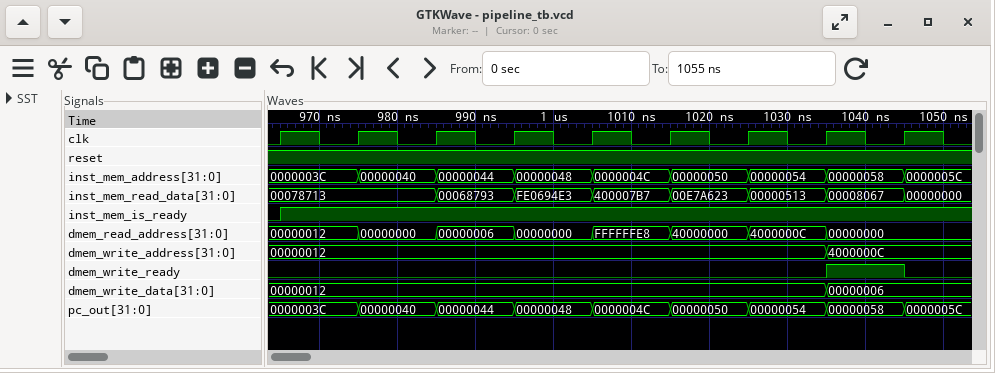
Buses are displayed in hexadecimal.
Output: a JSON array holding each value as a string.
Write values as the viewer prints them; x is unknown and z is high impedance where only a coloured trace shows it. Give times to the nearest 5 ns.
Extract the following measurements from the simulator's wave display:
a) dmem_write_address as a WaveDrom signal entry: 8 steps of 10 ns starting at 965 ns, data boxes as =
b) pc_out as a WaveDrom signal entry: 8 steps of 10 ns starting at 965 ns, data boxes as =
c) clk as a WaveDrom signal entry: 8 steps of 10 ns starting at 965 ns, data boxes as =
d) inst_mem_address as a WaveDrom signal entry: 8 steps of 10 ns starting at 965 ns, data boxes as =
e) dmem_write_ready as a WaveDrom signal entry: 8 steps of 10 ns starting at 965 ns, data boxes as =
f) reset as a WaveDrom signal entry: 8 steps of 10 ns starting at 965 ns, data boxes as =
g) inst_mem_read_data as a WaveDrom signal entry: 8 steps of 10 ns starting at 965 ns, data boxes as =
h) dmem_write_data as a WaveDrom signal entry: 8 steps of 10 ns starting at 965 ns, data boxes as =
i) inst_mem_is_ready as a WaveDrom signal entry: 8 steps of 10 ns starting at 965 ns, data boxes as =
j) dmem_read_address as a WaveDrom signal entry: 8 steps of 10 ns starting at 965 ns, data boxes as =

["{name: 'dmem_write_address', wave: '=......=', data: '00000012 4000000C'}", "{name: 'pc_out', wave: '========', data: '0000003C 00000040 00000044 00000048 0000004C 00000050 00000054 00000058'}", "{name: 'clk', wave: 'p.......'}", "{name: 'inst_mem_address', wave: '========', data: '0000003C 00000040 00000044 00000048 0000004C 00000050 00000054 00000058'}", "{name: 'dmem_write_ready', wave: '0......1'}", "{name: 'reset', wave: '1.......'}", "{name: 'inst_mem_read_data', wave: '=.======', data: '00078713 00068793 FE0694E3 400007B7 00E7A623 00000513 00008067'}", "{name: 'dmem_write_data', wave: '=......=', data: '00000012 00000006'}", "{name: 'inst_mem_is_ready', wave: '1.......'}", "{name: 'dmem_read_address', wave: '========', data: '00000012 00000000 00000006 00000000 FFFFFFE8 40000000 4000000C 00000000'}"]
